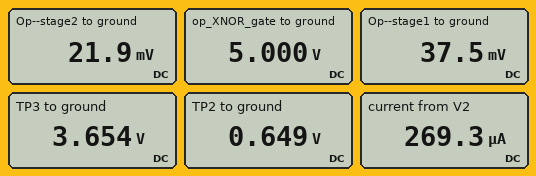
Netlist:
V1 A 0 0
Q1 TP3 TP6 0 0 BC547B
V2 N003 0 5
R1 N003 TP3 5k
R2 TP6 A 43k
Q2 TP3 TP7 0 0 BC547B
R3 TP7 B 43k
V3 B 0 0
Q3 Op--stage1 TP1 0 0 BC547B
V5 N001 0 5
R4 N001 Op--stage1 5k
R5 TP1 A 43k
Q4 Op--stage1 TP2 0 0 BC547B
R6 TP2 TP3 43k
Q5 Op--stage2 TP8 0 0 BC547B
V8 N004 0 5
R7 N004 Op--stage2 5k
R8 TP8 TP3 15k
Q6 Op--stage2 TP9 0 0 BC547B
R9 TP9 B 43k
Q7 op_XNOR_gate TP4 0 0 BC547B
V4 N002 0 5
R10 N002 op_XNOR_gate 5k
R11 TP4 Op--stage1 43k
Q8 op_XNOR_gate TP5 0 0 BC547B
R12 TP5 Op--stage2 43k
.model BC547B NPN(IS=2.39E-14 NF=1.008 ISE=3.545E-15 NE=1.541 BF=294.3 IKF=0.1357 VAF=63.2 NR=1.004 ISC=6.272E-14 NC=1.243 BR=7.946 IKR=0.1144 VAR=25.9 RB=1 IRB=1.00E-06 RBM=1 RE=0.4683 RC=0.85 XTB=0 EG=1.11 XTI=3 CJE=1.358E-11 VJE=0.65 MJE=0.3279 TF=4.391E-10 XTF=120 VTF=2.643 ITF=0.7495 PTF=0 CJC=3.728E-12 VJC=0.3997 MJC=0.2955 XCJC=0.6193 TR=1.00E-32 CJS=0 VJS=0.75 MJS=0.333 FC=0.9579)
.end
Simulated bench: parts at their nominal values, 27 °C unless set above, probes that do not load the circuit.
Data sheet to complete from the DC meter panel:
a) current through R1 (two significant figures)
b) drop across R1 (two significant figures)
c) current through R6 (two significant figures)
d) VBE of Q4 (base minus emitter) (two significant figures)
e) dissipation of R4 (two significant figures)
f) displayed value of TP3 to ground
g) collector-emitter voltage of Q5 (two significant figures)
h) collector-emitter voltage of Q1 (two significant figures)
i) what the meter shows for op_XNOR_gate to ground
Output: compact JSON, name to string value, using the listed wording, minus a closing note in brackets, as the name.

{"current through R1": "270 µA", "drop across R1": "1.3 V", "current through R6": "70 µA", "VBE of Q4 (base minus emitter)": "650 mV", "dissipation of R4": "4.9 mW", "displayed value of TP3 to ground": "3.654 V", "collector-emitter voltage of Q5": "22 mV", "collector-emitter voltage of Q1": "3.7 V", "what the meter shows for op_XNOR_gate to ground": "5.000 V"}
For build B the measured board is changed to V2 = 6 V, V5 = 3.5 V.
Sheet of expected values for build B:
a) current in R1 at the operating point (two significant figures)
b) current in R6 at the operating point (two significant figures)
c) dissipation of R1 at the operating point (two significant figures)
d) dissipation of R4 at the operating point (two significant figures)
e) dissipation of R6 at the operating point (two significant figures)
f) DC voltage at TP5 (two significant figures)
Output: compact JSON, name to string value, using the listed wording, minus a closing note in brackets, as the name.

{"current in R1 at the operating point": "330 µA", "current in R6 at the operating point": "86 µA", "dissipation of R1 at the operating point": "550 µW", "dissipation of R4 at the operating point": "2.4 mW", "dissipation of R6 at the operating point": "320 µW", "DC voltage at TP5": "20 mV"}
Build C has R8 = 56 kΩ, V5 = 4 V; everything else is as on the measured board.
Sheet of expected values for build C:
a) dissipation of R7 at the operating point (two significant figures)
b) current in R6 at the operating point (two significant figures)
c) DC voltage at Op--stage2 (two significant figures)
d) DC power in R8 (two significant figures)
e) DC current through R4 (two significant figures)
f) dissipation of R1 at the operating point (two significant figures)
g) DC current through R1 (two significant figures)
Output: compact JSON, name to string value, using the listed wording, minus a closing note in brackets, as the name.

{"dissipation of R7 at the operating point": "4.9 mW", "current in R6 at the operating point": "84 µA", "DC voltage at Op--stage2": "39 mV", "DC power in R8": "230 µW", "DC current through R4": "790 µA", "dissipation of R1 at the operating point": "110 µW", "DC current through R1": "150 µA"}
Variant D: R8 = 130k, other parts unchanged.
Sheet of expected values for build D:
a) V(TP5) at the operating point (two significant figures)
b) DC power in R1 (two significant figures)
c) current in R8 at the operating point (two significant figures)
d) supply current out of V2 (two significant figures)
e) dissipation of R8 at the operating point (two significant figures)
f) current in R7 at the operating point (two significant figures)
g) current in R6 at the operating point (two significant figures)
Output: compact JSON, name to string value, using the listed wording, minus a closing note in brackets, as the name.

{"V(TP5) at the operating point": "57 mV", "DC power in R1": "68 µW", "current in R8 at the operating point": "29 µA", "supply current out of V2": "120 µA", "dissipation of R8 at the operating point": "110 µW", "current in R7 at the operating point": "990 µA", "current in R6 at the operating point": "88 µA"}
